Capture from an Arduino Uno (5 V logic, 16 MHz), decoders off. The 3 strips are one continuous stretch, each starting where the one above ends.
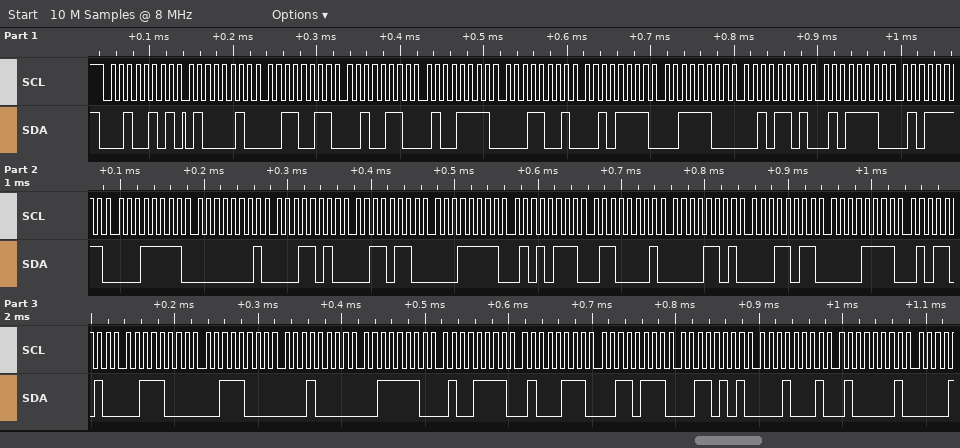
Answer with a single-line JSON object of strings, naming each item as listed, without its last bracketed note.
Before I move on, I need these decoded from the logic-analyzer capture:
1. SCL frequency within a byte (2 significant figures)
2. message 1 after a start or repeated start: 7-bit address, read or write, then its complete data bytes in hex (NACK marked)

{"SCL frequency within a byte": "100 kHz", "message 1 after a start or repeated start: 7-bit address, read or write, then its complete data bytes in hex": "0x12 read: 42 33 26 4F 19 2F 3C 2D 5E 5F 1F 01 1A 36 1F 57 61 0D 1B 0F 5A 38 38 10 3E 4F 47 37 35 11 41"}
